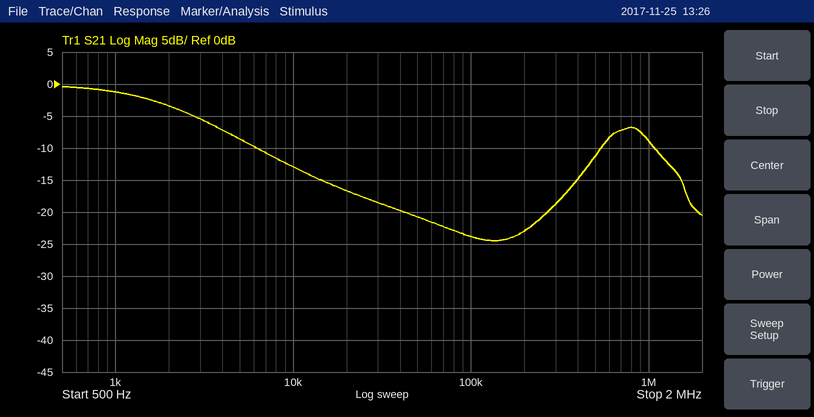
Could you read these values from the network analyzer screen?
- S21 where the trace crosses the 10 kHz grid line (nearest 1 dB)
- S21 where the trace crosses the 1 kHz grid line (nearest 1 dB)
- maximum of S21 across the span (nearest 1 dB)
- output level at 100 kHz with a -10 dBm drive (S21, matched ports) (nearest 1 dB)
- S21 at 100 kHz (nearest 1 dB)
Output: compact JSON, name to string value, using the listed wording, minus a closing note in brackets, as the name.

{"S21 where the trace crosses the 10 kHz grid line": "-13 dB", "S21 where the trace crosses the 1 kHz grid line": "-1 dB", "maximum of S21 across the span": "0 dB", "output level at 100 kHz with a -10 dBm drive (S21, matched ports)": "-34 dBm", "S21 at 100 kHz": "-24 dB"}
